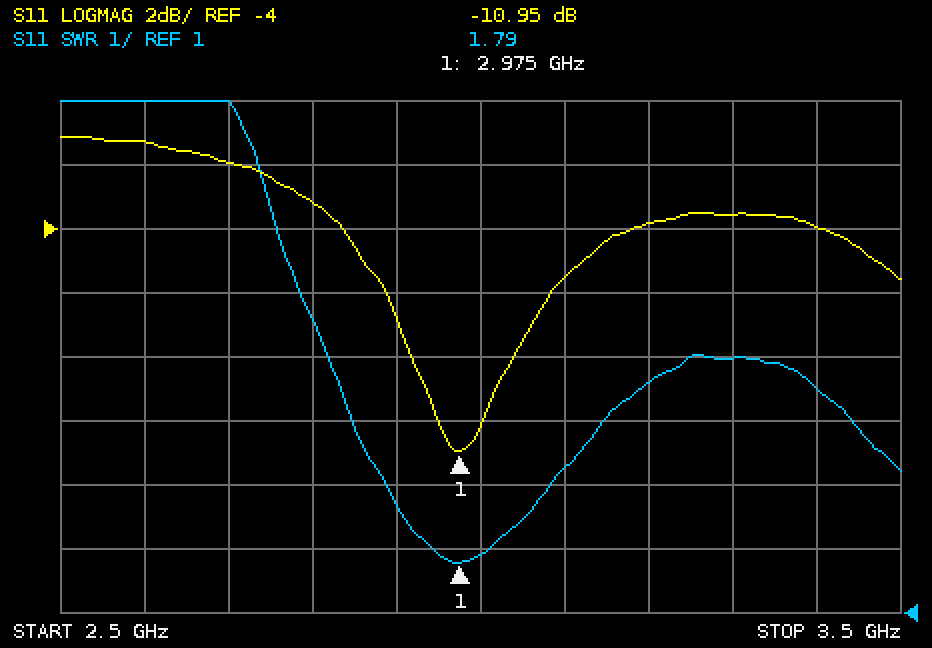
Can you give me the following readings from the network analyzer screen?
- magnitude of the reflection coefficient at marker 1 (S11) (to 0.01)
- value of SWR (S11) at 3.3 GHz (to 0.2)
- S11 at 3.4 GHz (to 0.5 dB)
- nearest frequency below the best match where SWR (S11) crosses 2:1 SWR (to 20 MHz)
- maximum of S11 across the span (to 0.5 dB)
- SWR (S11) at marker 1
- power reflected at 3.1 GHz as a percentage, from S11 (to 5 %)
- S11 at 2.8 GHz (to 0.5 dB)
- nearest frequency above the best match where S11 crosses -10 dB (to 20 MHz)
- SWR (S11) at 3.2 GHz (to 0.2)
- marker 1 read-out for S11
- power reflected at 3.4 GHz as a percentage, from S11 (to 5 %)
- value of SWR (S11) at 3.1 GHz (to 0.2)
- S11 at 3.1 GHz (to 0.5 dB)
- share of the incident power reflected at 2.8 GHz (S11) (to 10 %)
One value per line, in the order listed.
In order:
0.28
5.0
-4.0 dB
2.94 GHz
-1.0 dB
1.79
30 %
-3.0 dB
3.00 GHz
4.6
-10.95 dB
40 %
3.2
-5.5 dB
50 %
